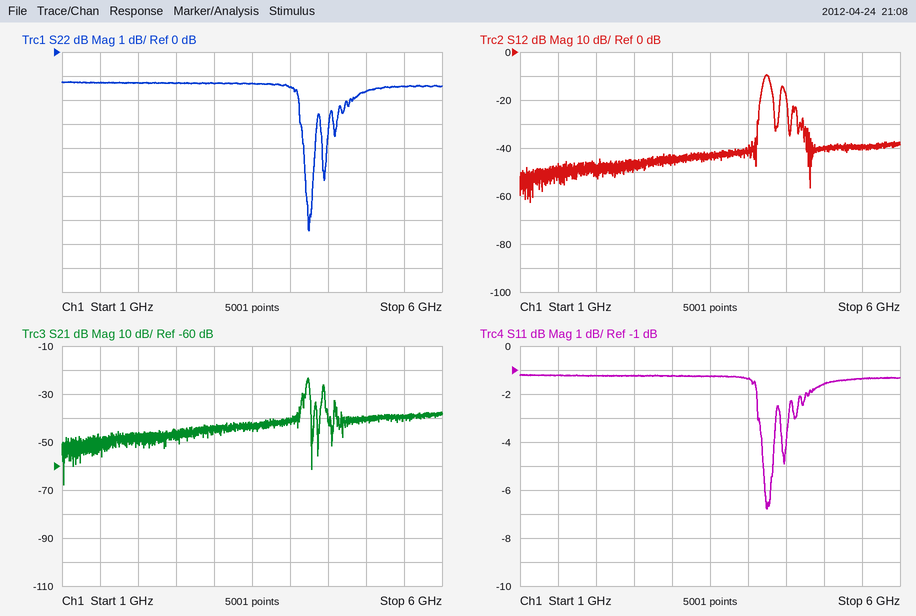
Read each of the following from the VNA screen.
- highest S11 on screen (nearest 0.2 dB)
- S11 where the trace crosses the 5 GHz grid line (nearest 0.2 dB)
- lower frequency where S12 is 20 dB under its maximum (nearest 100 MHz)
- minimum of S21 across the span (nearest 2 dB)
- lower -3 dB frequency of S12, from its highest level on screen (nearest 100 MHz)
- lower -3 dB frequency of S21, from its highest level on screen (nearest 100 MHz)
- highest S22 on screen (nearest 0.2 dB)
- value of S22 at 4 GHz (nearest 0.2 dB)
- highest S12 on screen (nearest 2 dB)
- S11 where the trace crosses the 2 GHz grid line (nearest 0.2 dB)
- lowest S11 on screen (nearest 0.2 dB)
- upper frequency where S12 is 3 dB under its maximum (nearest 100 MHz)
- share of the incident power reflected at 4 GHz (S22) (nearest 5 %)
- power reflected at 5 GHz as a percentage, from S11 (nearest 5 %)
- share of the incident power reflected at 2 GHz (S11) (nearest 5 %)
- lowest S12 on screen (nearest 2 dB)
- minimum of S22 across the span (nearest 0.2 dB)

-1.2 dB
-1.6 dB
4.1 GHz
-68 dB
4.2 GHz
4.2 GHz
-1.2 dB
-1.4 dB
-10 dB
-1.2 dB
-6.8 dB
4.3 GHz
70 %
70 %
75 %
-62 dB
-7.4 dB
